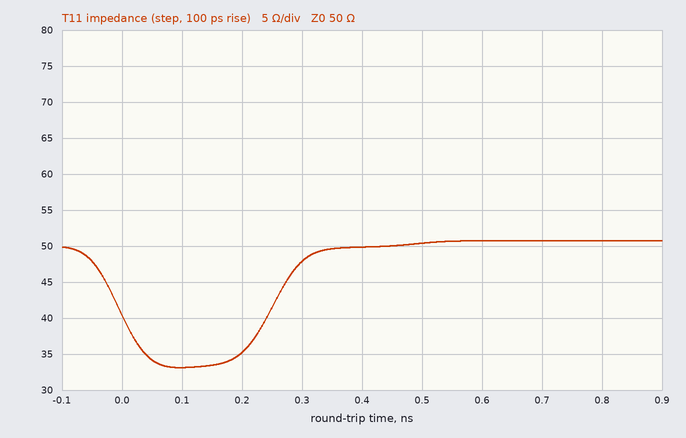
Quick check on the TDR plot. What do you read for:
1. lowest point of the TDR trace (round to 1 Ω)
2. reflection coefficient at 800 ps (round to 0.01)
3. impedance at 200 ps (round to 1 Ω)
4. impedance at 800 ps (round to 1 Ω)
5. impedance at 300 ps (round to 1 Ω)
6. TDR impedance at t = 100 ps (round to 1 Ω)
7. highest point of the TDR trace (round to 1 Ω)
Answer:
33 Ω
+0.01
35 Ω
51 Ω
48 Ω
33 Ω
51 Ω
